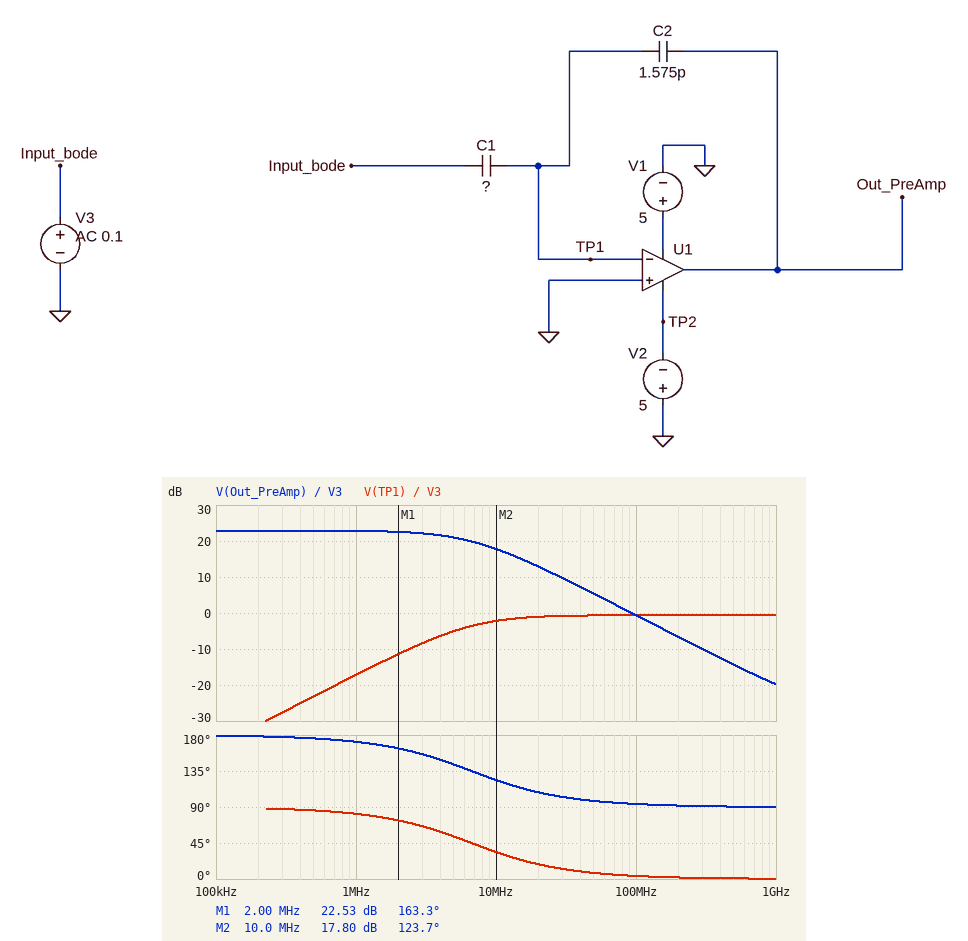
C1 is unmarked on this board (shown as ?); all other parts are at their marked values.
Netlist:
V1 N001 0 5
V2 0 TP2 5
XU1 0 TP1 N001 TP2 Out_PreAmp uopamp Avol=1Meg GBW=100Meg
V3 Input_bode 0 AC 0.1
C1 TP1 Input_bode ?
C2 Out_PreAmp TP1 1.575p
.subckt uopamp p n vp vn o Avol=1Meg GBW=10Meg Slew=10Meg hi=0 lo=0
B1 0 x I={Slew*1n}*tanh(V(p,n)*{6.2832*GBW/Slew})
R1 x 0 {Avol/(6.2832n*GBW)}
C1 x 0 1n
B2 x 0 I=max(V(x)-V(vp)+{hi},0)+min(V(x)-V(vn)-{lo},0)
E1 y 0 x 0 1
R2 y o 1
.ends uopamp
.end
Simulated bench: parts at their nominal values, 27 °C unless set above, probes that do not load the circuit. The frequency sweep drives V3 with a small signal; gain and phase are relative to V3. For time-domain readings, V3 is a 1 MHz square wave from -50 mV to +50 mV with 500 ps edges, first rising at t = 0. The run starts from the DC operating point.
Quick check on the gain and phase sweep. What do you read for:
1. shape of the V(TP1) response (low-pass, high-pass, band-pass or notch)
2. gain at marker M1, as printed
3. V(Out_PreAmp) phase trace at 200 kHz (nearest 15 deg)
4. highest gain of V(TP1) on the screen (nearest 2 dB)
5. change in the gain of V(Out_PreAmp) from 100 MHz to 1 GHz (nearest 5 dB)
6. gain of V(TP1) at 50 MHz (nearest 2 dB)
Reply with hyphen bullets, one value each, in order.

- high-pass
- 22.53 dB
- 180 deg
- 0 dB
- -20 dB
- 0 dB
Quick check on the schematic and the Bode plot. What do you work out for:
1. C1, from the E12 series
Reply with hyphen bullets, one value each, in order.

- 22 pF
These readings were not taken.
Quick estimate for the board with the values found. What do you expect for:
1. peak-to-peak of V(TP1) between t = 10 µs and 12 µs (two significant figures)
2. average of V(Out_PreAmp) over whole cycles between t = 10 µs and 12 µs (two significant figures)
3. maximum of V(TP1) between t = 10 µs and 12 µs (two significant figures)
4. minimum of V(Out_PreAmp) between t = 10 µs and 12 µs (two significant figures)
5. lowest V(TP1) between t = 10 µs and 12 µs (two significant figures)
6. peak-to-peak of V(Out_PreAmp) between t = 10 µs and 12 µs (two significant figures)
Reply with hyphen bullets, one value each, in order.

- 190 mV
- -700 mV
- 93 mV
- -1.4 V
- -93 mV
- 1.4 V
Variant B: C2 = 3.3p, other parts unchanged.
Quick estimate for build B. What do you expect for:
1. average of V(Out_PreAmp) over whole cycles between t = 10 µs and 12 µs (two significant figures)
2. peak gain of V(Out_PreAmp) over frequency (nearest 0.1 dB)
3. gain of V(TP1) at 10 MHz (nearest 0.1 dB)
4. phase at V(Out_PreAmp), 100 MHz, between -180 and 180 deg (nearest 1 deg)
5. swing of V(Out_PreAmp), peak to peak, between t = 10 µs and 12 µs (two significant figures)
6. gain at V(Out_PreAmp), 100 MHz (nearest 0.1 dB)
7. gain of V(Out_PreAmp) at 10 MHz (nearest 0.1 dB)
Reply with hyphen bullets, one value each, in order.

- -330 mV
- 16.5 dB
- -5.5 dB
- 97 deg
- 670 mV
- -1.3 dB
- 14.5 dB
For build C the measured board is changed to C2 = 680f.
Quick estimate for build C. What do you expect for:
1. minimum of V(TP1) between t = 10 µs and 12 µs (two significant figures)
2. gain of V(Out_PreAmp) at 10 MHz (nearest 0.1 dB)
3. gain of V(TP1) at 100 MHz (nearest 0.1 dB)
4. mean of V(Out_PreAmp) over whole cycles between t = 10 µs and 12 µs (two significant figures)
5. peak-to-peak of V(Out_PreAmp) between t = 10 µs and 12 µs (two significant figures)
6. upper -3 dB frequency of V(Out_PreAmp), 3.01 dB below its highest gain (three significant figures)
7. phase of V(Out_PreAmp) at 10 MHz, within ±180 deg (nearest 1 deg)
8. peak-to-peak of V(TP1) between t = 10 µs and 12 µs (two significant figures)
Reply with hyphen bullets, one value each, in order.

- -97 mV
- 19.4 dB
- -0.3 dB
- -1.6 V
- 3.2 V
- 3.00 MHz
- 107 deg
- 190 mV
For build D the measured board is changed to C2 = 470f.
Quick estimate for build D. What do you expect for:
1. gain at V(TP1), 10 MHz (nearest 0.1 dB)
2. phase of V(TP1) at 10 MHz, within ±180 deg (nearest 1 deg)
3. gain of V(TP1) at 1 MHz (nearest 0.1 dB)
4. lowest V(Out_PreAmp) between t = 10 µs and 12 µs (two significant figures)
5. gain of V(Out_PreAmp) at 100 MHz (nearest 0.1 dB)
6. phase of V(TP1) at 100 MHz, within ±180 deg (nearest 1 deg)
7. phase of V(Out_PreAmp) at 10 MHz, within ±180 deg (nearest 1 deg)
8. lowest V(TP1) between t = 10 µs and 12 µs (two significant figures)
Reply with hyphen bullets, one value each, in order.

- -0.4 dB
- 12 deg
- -7.5 dB
- -4.5 V
- -0.2 dB
- 1 deg
- 102 deg
- -94 mV
